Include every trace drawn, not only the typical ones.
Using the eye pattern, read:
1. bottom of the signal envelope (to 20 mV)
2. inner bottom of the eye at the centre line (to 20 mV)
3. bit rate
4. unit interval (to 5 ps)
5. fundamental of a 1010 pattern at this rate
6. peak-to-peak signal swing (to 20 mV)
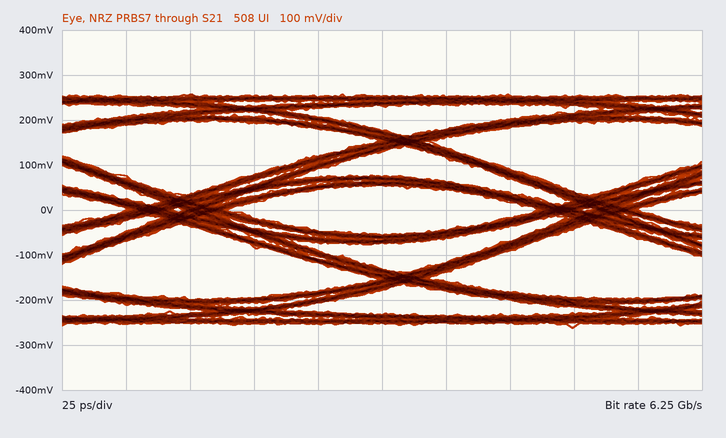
-260 mV
-60 mV
6.25 Gb/s
160 ps
3.125 GHz
520 mV
